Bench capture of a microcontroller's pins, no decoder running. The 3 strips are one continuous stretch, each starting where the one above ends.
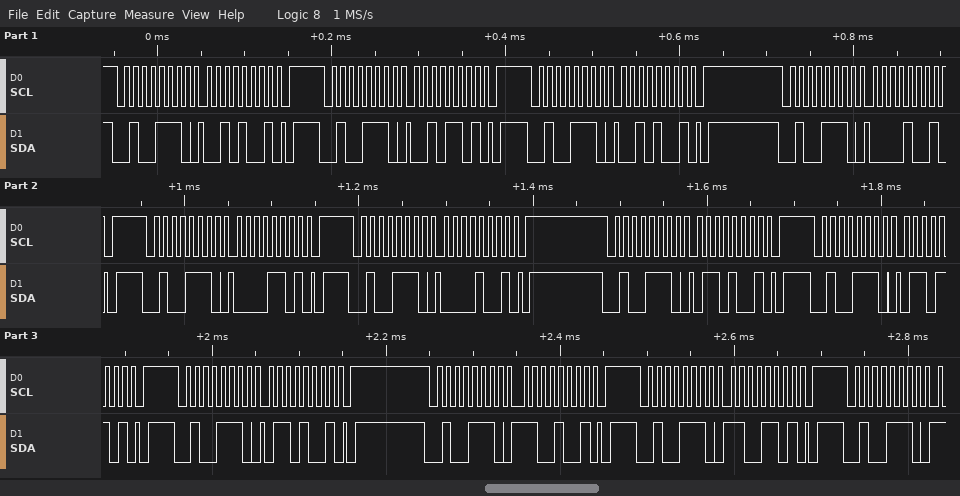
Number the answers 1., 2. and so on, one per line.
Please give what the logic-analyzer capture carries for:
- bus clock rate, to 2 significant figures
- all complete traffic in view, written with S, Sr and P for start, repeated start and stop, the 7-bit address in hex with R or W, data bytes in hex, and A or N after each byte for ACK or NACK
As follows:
1. 100 kHz
2. S 27W A 29 A P S 27W A 2D A P S 27W A 29 A P S 27W A 09 A P S 27W A 0D A P S 27W A 09 A P S 27W A 69 A P S 27W A 6D A P S 27W A 69 A P S 27W A C9 A P S 27W A CD A P S 27W A
